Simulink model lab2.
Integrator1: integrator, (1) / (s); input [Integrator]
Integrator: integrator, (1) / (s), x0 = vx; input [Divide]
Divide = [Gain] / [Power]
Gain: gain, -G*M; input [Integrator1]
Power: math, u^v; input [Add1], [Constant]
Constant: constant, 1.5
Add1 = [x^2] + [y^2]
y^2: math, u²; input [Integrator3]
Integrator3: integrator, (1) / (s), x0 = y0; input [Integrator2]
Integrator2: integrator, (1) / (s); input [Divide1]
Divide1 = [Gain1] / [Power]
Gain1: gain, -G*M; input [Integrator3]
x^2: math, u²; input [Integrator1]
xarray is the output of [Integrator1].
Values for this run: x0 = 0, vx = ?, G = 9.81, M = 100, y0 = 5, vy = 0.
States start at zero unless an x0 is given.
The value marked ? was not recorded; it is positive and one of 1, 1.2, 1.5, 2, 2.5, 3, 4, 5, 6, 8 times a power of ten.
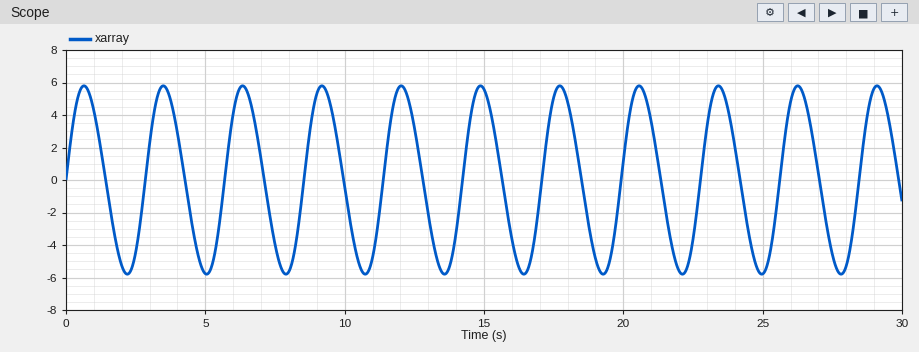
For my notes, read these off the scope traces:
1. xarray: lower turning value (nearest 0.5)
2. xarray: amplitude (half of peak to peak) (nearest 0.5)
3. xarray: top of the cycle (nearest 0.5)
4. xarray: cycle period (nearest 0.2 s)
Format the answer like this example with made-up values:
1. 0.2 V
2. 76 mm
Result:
1. -6.0
2. 6.0
3. 6.0
4. 2.8 s
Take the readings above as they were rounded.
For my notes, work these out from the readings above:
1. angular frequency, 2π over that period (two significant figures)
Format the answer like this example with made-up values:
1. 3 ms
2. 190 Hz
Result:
1. 2.2 rad/s
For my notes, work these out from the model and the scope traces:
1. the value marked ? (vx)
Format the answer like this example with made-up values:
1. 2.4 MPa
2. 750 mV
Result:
1. 15
